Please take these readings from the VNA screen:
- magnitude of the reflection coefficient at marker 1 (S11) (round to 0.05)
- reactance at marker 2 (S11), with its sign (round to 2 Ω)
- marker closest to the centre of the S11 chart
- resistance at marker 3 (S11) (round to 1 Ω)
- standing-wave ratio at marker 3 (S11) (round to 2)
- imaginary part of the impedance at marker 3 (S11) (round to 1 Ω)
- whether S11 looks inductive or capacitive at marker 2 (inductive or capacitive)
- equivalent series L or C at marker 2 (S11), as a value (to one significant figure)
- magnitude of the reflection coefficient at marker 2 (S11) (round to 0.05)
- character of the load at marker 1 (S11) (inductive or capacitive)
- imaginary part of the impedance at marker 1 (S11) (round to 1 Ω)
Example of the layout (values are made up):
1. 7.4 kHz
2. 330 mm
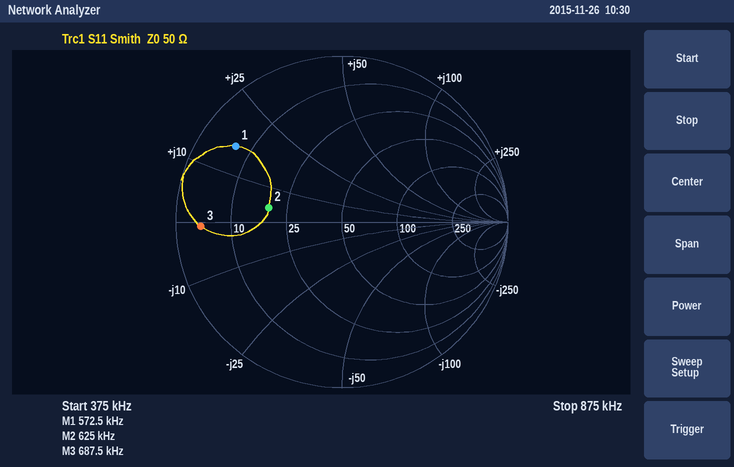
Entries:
1. 0.80
2. +4 Ω
3. marker 2
4. 4 Ω
5. 12
6. -1 Ω
7. inductive
8. 1 µH
9. 0.45
10. inductive
11. +16 Ω
